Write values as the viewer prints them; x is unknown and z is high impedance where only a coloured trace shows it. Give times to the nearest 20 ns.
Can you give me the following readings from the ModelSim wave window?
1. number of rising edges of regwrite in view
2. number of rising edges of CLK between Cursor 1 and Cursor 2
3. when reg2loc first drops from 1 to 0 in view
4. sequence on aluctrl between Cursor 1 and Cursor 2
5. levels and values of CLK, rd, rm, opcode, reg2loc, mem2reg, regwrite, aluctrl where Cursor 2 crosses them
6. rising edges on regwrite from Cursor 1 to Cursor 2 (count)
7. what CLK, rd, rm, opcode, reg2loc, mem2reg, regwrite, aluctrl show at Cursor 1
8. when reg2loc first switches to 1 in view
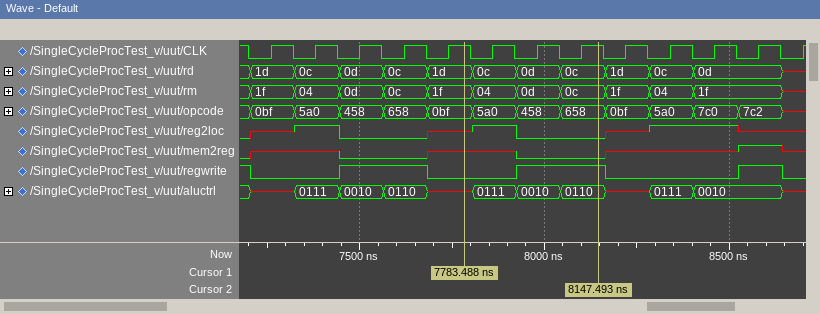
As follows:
3
3
7440 ns
x, 0111, 0010, 0110
CLK=1, rd=0c, rm=0c, opcode=658, reg2loc=0, mem2reg=0, regwrite=1, aluctrl=0110
1
CLK=1, rd=1d, rm=1f, opcode=0bf, reg2loc=x, mem2reg=x, regwrite=0, aluctrl=x
7320 ns
